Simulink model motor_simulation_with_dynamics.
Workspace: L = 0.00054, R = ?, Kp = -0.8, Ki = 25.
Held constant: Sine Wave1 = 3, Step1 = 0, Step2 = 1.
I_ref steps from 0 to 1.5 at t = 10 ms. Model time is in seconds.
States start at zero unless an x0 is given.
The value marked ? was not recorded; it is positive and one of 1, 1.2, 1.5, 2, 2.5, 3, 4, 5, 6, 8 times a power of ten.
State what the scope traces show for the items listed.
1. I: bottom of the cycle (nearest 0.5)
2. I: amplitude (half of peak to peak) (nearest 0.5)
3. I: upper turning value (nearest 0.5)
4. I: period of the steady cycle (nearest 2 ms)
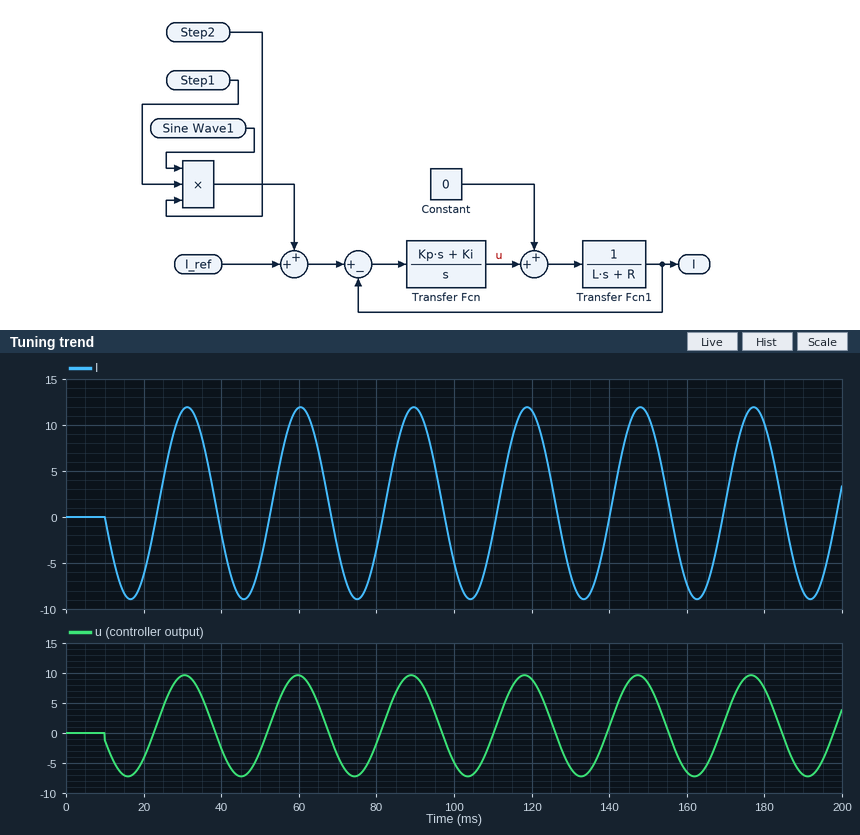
-9.0
10.5
12.0
30 ms
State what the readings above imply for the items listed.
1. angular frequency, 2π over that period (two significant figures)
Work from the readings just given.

0.21 rad/ms
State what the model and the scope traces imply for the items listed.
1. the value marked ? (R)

0.8
